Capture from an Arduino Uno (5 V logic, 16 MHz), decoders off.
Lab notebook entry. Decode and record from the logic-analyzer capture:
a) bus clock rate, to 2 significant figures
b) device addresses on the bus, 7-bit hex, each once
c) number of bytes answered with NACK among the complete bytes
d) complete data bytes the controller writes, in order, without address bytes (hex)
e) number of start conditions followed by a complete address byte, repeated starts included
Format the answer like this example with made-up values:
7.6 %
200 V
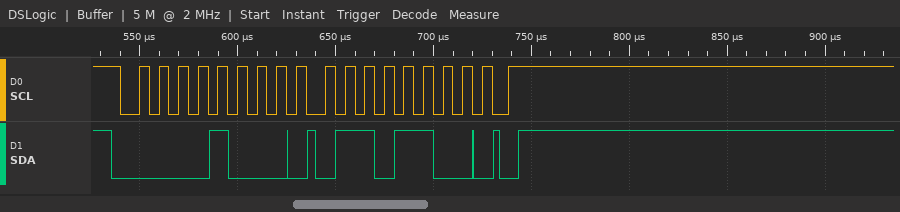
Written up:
100 kHz
0x04
0
6C
1
